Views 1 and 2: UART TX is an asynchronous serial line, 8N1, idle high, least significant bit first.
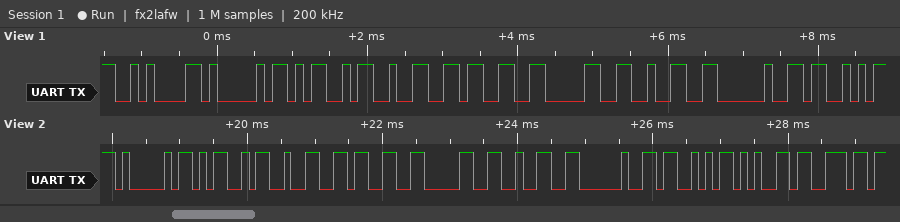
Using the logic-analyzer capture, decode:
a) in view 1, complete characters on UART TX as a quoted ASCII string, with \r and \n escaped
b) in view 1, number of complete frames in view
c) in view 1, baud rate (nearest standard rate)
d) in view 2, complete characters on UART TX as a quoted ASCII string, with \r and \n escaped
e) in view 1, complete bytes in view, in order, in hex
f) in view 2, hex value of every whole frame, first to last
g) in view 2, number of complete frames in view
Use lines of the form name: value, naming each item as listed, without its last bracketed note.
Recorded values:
in view 1, complete characters on UART TX as a quoted ASCII string, with \r and \n escaped: "\nAM2302 S"
in view 1, number of complete frames in view: 9
in view 1, baud rate: 9600 baud
in view 2, complete characters on UART TX as a quoted ASCII string, with \r and \n escaped: "AM2302 Sen"
in view 1, complete bytes in view, in order, in hex: 0A 41 4D 32 33 30 32 20 53
in view 2, hex value of every whole frame, first to last: 0x41 0x4D 0x32 0x33 0x30 0x32 0x20 0x53 0x65 0x6E
in view 2, number of complete frames in view: 10
